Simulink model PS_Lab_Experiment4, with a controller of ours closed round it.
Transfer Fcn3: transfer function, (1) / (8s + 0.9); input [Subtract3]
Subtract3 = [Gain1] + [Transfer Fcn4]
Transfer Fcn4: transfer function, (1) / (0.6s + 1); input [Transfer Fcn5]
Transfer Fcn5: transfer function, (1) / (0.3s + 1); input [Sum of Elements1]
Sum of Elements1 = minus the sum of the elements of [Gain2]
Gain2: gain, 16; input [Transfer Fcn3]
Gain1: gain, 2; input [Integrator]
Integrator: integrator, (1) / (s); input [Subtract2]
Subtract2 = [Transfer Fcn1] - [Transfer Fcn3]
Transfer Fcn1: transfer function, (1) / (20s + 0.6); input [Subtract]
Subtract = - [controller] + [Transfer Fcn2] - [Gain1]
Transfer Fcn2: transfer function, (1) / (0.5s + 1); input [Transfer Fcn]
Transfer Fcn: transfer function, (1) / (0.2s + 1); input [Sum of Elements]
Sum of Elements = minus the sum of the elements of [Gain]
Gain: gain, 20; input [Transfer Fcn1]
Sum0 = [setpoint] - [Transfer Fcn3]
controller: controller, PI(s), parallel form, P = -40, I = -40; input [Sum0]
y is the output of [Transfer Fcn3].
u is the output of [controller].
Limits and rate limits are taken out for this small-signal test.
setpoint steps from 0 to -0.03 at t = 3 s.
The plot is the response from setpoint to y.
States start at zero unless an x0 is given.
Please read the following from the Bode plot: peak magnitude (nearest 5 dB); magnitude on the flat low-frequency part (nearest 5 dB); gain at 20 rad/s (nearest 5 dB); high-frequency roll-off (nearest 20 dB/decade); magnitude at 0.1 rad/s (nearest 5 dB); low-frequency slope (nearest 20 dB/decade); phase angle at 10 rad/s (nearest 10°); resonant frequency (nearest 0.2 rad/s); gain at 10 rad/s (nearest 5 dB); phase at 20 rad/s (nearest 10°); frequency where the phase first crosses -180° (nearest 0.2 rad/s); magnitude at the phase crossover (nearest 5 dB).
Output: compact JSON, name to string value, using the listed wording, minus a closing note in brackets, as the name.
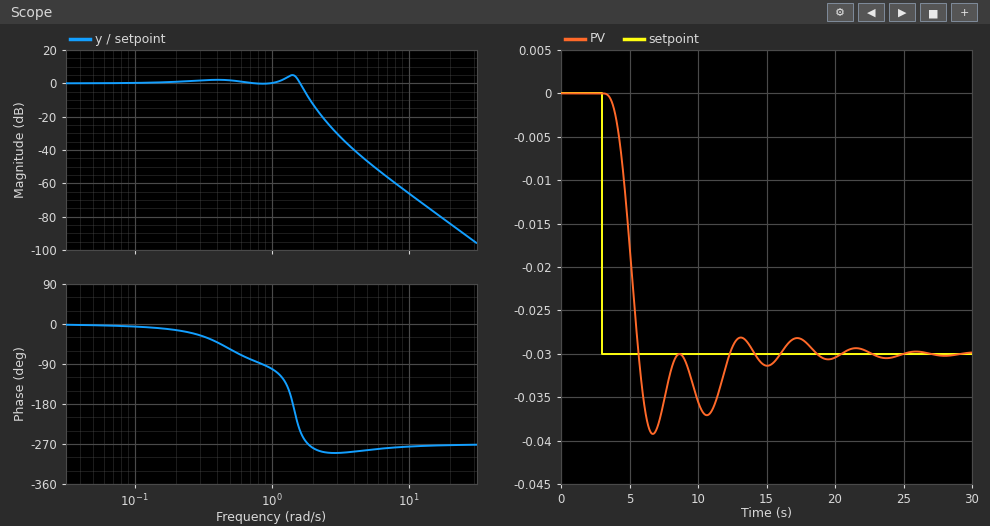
{"peak magnitude": "5 dB", "magnitude on the flat low-frequency part": "0 dB", "gain at 20 rad/s": "-85 dB", "high-frequency roll-off": "-60 dB/decade", "magnitude at 0.1 rad/s": "0 dB", "low-frequency slope": "0 dB/decade", "phase angle at 10 rad/s": "-280°", "resonant frequency": "1.4 rad/s", "gain at 10 rad/s": "-65 dB", "phase at 20 rad/s": "-270°", "frequency where the phase first crosses -180°": "1.4 rad/s", "magnitude at the phase crossover": "5 dB"}
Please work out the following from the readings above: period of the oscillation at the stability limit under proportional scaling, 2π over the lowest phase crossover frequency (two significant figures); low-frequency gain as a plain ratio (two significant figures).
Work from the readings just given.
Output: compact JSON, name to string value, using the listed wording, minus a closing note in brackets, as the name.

{"period of the oscillation at the stability limit under proportional scaling, 2π over the lowest phase crossover frequency": "4.5 s", "low-frequency gain as a plain ratio": "1.0"}
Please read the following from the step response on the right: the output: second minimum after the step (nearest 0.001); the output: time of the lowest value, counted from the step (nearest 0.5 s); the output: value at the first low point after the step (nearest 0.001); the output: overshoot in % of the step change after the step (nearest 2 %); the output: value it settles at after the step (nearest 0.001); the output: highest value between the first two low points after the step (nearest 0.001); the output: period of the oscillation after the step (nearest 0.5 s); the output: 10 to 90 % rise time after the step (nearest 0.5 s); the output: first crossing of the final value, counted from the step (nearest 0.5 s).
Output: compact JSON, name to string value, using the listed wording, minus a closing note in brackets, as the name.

{"the output: second minimum after the step": "-0.037", "the output: time of the lowest value, counted from the step": "3.5 s", "the output: value at the first low point after the step": "-0.039", "the output: overshoot in % of the step change after the step": "30 %", "the output: value it settles at after the step": "-0.030", "the output: highest value between the first two low points after the step": "-0.030", "the output: period of the oscillation after the step": "4.0 s", "the output: 10 to 90 % rise time after the step": "1.5 s", "the output: first crossing of the final value, counted from the step": "2.5 s"}
